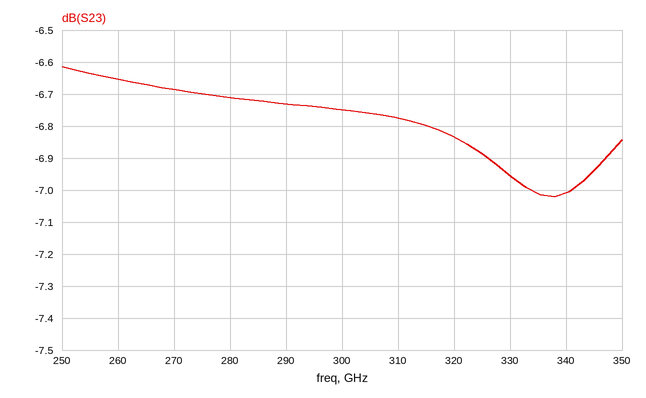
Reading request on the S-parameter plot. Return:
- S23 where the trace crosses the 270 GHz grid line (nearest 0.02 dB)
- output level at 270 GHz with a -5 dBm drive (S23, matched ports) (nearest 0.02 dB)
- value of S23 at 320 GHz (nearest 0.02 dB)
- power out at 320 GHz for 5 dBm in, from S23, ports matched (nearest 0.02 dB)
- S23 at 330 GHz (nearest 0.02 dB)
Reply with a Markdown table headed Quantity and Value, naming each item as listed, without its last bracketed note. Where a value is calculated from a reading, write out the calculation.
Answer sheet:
| Quantity | Value |
|---|---|
| S23 where the trace crosses the 270 GHz grid line | -6.68 dB |
| output level at 270 GHz with a -5 dBm drive (S23, matched ports) | -5 dBm + (-6.68 dB) = -11.68 dBm |
| value of S23 at 320 GHz | -6.84 dB |
| power out at 320 GHz for 5 dBm in, from S23, ports matched | 5 dBm + (-6.84 dB) = -1.84 dBm |
| S23 at 330 GHz | -6.96 dB |
